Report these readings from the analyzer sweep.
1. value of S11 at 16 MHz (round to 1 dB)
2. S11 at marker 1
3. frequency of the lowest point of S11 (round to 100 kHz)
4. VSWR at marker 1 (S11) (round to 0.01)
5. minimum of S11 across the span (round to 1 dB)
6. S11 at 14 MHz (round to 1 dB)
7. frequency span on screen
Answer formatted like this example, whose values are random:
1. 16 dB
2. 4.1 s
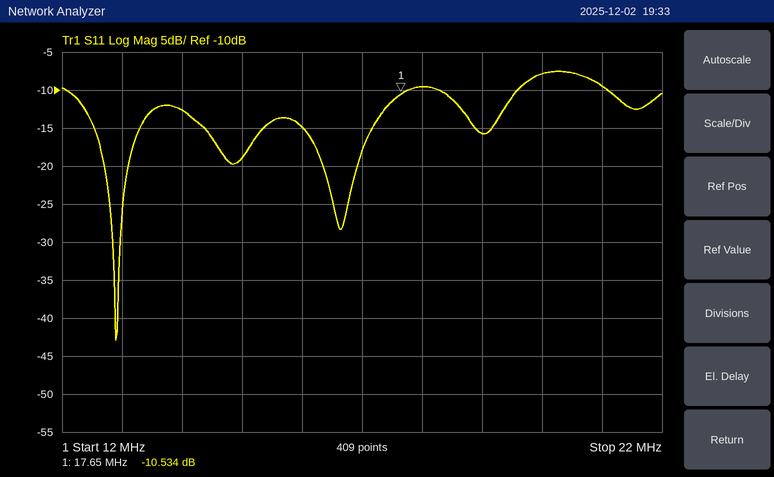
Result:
1. -15 dB
2. -10.534 dB
3. 12.9 MHz
4. 1.85
5. -43 dB
6. -13 dB
7. 10 MHz
